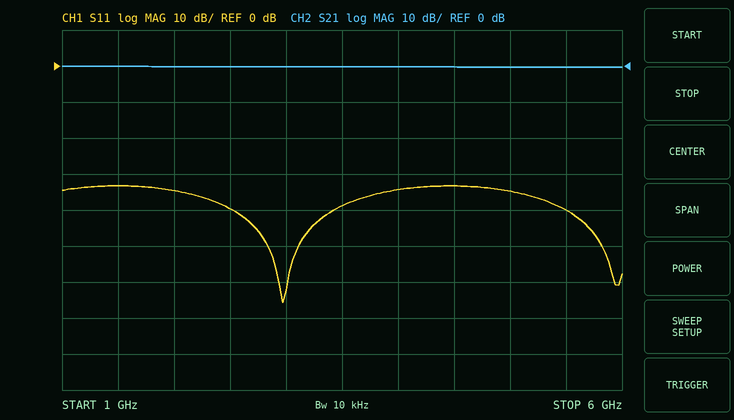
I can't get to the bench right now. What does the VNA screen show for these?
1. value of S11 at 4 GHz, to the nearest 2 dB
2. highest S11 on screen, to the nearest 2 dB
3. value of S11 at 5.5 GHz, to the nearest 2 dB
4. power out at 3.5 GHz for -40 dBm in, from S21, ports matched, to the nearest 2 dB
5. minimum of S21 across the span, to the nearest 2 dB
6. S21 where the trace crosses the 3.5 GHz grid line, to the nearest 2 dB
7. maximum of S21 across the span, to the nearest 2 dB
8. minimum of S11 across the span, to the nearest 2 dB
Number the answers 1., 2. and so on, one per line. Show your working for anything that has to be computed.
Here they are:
1. -34 dB
2. -34 dB
3. -40 dB
4. -40 dBm + (0 dB) = -40 dBm
5. 0 dB
6. 0 dB
7. 0 dB
8. -66 dB
